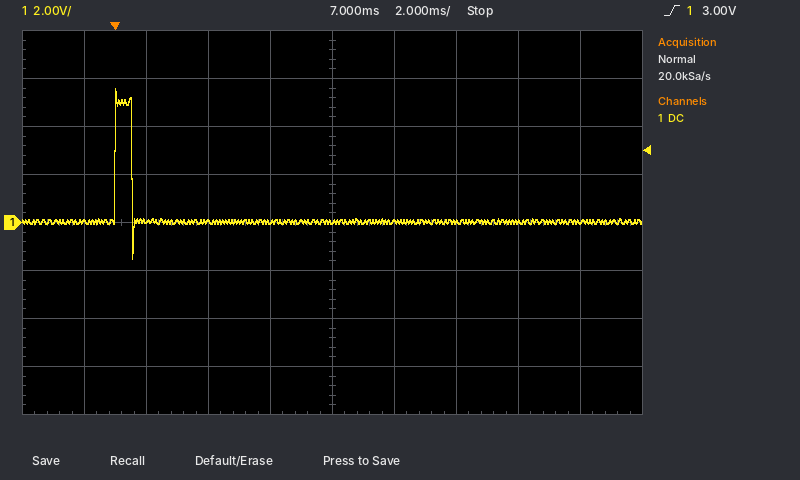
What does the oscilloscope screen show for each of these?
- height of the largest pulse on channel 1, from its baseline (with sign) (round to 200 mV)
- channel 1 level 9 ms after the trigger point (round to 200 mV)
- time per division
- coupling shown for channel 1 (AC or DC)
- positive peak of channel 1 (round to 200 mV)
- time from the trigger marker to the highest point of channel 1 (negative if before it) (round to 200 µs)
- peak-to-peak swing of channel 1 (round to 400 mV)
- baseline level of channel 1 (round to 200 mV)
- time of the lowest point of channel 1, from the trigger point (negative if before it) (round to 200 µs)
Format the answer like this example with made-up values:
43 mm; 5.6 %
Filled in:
+5.6 V; 0.0 V; 2 ms; DC; 5.6 V; 0.0 ms; 7.2 V; 0.0 V; +600 µs
